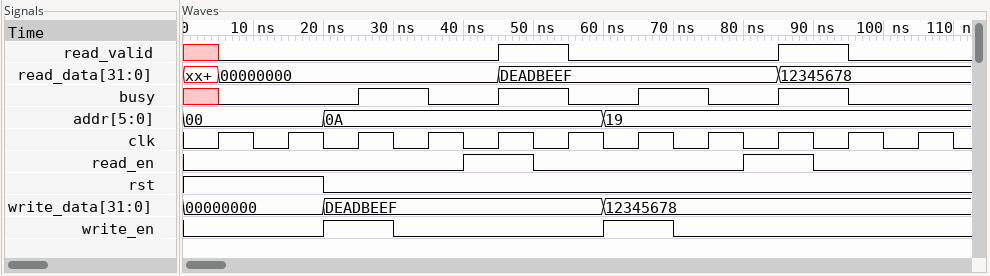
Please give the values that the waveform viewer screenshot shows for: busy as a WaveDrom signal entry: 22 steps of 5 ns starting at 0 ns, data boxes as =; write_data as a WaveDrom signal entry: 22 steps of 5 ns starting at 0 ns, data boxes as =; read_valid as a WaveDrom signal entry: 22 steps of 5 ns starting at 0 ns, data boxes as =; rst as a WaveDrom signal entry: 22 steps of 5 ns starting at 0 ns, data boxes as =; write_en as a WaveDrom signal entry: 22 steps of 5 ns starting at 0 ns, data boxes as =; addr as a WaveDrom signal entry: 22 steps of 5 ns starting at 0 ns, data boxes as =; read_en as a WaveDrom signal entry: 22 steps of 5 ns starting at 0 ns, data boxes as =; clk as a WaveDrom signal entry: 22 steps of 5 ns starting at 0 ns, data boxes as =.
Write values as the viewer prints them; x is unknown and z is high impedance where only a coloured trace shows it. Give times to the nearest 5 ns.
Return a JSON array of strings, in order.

["{name: 'busy', wave: 'x0...1.0.1.0.1.0.1.0..'}", "{name: 'write_data', wave: '=...=.......=.........', data: '00000000 DEADBEEF 12345678'}", "{name: 'read_valid', wave: 'x0.......1.0.....1.0..'}", "{name: 'rst', wave: '1...0.................'}", "{name: 'write_en', wave: '0...1.0.....1.0.......'}", "{name: 'addr', wave: '=...=.......=.........', data: '00 0A 19'}", "{name: 'read_en', wave: '0.......1.0.....1.0...'}", "{name: 'clk', wave: '0101010101010101010101'}"]
